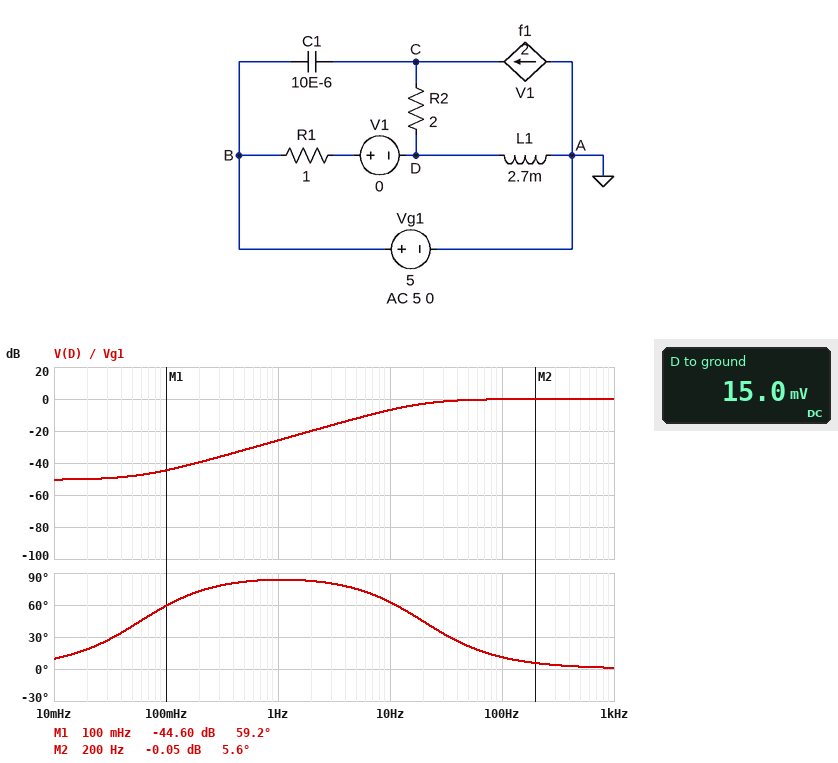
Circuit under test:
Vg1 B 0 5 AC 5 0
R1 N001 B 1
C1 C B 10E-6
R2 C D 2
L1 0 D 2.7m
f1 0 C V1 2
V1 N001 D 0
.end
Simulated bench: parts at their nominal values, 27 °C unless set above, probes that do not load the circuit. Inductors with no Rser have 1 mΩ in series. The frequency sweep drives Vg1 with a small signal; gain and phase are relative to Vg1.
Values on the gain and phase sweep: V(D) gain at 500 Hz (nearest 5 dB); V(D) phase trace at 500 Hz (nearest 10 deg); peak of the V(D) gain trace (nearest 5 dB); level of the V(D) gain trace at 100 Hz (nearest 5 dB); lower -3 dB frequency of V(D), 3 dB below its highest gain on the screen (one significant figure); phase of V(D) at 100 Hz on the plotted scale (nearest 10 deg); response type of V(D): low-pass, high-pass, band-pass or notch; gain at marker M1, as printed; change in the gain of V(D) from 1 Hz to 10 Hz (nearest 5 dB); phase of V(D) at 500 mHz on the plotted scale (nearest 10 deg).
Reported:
0 dB
0 deg
0 dB
0 dB
20 Hz
10 deg
high-pass
-44.60 dB
20 dB
80 deg
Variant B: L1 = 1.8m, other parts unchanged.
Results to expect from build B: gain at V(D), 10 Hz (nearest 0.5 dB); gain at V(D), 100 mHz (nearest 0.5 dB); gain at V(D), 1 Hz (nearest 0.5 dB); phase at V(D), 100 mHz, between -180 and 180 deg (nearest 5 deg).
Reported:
-10.0 dB
-47.0 dB
-29.5 dB
50 deg
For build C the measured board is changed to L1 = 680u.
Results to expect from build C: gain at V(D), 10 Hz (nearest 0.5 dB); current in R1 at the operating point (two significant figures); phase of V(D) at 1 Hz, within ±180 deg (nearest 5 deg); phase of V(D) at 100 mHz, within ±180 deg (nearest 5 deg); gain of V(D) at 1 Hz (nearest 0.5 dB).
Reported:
-18.0 dB
5.0 A
75 deg
25 deg
-37.5 dB
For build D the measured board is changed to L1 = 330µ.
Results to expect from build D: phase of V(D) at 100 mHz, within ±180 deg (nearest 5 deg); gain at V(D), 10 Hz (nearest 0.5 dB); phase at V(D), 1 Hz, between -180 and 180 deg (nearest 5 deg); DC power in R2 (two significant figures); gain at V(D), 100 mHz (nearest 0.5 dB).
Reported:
10 deg
-24.0 dB
65 deg
200 W
-50.5 dB
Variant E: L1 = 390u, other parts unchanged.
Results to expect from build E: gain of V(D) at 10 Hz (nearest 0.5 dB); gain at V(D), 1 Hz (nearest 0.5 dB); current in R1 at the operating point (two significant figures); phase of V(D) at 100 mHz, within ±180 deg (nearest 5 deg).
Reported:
-22.5 dB
-42.0 dB
5.0 A
15 deg
